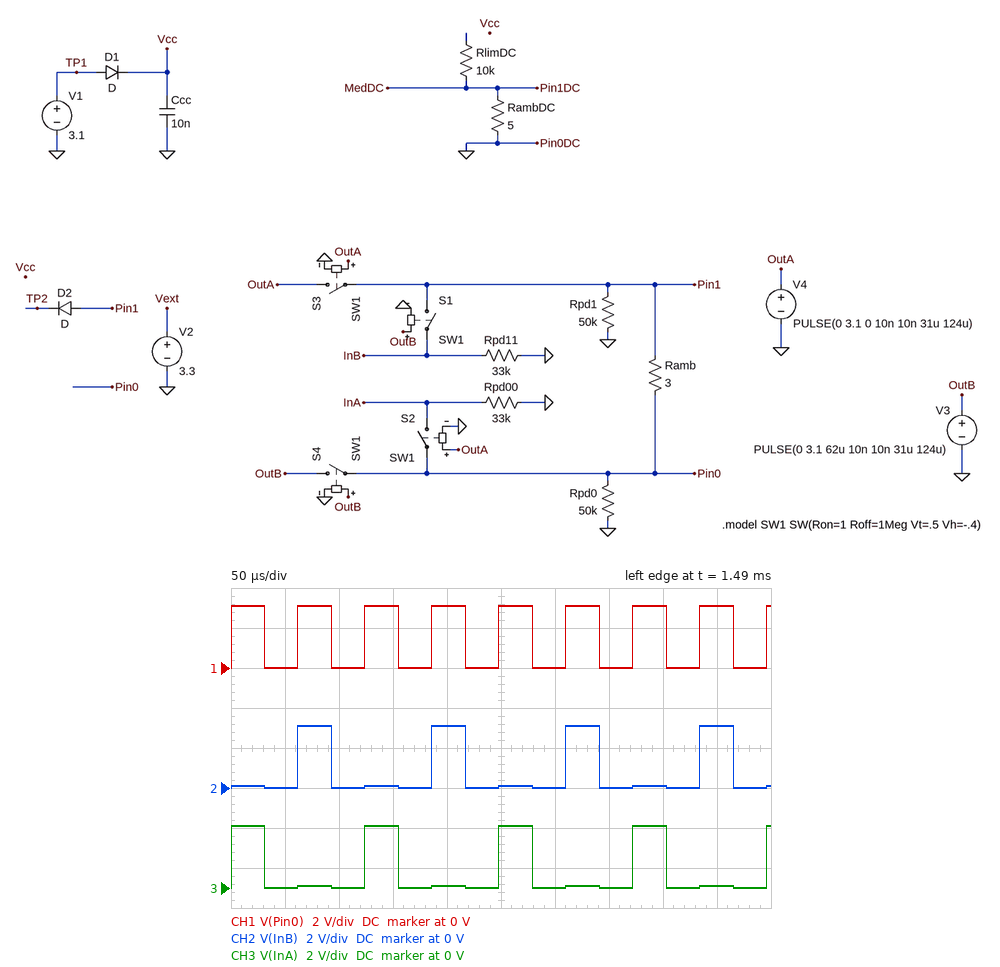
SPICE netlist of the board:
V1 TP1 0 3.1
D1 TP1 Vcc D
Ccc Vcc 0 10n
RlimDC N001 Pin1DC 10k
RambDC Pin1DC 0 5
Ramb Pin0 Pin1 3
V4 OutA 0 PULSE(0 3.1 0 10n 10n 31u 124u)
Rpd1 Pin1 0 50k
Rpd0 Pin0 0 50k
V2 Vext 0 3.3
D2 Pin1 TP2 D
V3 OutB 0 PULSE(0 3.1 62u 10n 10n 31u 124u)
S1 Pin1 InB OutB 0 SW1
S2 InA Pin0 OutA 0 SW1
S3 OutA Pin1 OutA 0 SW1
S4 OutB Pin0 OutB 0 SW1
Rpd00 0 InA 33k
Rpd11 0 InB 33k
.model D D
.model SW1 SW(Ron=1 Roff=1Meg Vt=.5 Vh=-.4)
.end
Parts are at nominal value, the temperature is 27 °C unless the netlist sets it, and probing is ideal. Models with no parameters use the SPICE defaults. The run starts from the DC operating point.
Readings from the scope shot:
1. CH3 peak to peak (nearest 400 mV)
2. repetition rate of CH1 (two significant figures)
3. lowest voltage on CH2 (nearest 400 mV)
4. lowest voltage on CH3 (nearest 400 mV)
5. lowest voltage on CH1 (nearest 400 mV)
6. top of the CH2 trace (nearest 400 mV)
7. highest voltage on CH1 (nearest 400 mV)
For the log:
3.2 V
16 kHz
0 V
0 V
0 V
3.2 V
3.2 V
